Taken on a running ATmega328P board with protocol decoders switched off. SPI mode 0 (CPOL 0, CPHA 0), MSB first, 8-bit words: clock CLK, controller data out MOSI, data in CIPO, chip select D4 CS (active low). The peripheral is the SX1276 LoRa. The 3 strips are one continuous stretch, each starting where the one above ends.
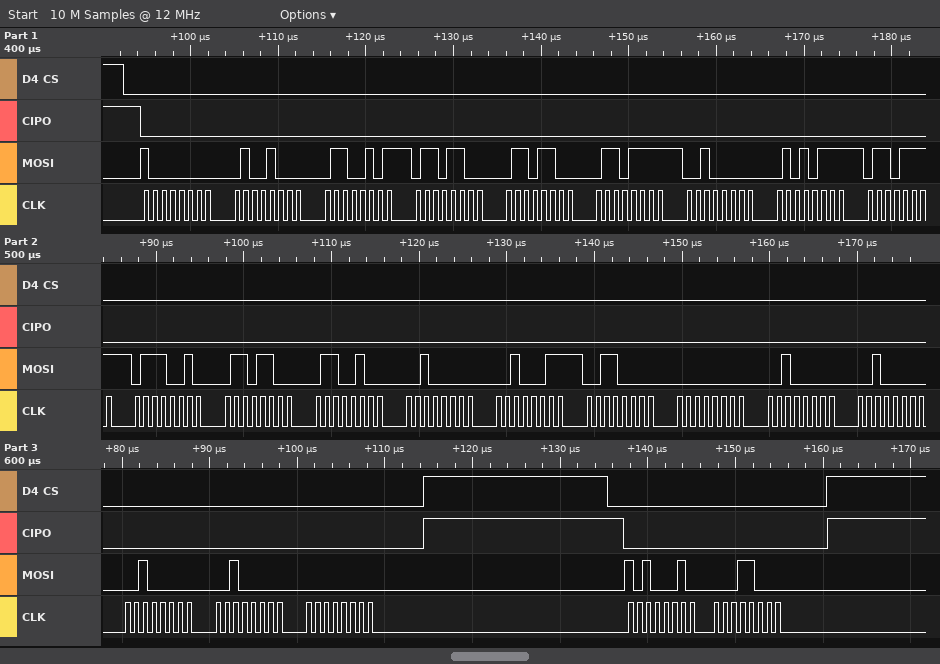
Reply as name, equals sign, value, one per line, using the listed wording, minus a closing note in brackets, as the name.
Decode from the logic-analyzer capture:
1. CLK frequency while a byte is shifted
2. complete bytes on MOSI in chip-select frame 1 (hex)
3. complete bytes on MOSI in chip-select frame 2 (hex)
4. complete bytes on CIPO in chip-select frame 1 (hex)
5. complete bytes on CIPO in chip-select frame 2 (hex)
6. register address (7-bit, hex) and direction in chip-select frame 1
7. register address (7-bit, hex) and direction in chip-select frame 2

CLK frequency while a byte is shifted = 1 MHz
complete bytes on MOSI in chip-select frame 1 = 80 48 65 6C 6C 6F 20 57 6F 72 6C 64 20 23 30 00 20 20 20 20 00
complete bytes on MOSI in chip-select frame 2 = A2 18
complete bytes on CIPO in chip-select frame 1 = 00 00 00 00 00 00 00 00 00 00 00 00 00 00 00 00 00 00 00 00 00
complete bytes on CIPO in chip-select frame 2 = 00 00
register address (7-bit, hex) and direction in chip-select frame 1 = 0x00 write
register address (7-bit, hex) and direction in chip-select frame 2 = 0x22 write
